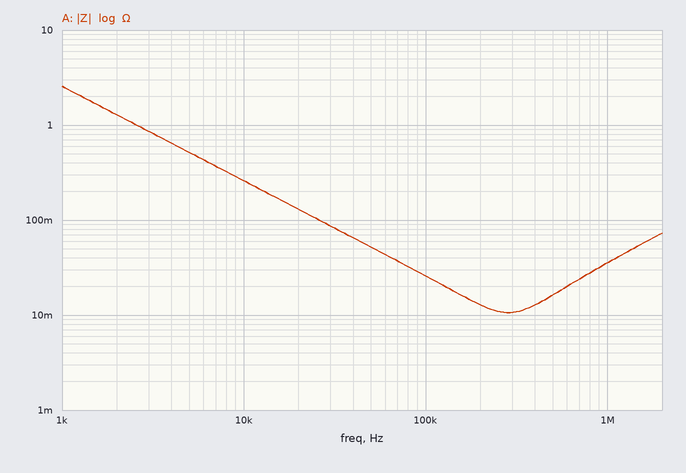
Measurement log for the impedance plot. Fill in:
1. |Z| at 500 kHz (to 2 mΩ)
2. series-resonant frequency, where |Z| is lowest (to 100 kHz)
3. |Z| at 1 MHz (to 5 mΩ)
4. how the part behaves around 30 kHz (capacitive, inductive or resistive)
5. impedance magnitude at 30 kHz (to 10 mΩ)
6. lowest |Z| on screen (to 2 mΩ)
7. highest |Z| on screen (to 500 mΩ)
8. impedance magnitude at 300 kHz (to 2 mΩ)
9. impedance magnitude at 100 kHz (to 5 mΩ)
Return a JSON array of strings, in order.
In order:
["16 mΩ", "300 kHz", "35 mΩ", "capacitive", "90 mΩ", "10 mΩ", "2.5 Ω", "10 mΩ", "25 mΩ"]
